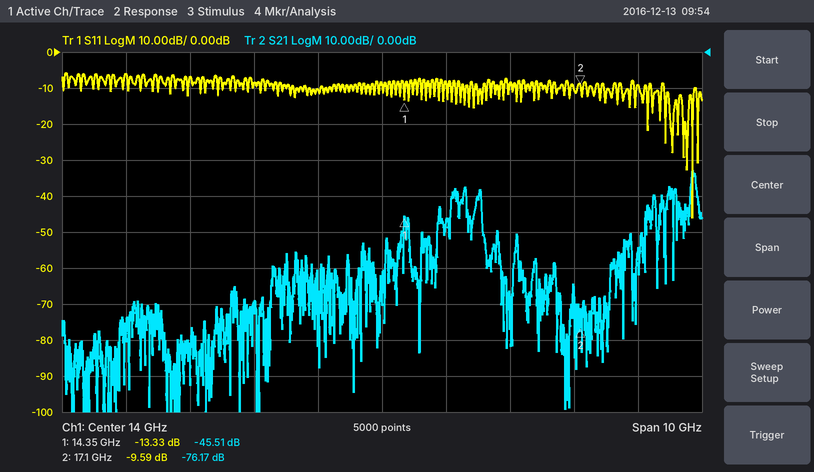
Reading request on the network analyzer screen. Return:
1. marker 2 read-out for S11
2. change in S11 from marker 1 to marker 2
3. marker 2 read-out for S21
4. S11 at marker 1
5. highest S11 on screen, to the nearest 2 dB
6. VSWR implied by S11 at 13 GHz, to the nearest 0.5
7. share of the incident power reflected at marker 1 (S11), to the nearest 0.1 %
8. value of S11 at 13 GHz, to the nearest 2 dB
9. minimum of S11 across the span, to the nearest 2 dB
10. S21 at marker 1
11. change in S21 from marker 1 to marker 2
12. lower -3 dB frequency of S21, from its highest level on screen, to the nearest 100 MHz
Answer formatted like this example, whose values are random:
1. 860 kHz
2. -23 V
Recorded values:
1. -9.59 dB
2. 3.74 dB
3. -76.17 dB
4. -13.33 dB
5. -6 dB
6. 2.0
7. 4.6 %
8. -10 dB
9. -46 dB
10. -45.51 dB
11. -30.66 dB
12. 18.8 GHz
